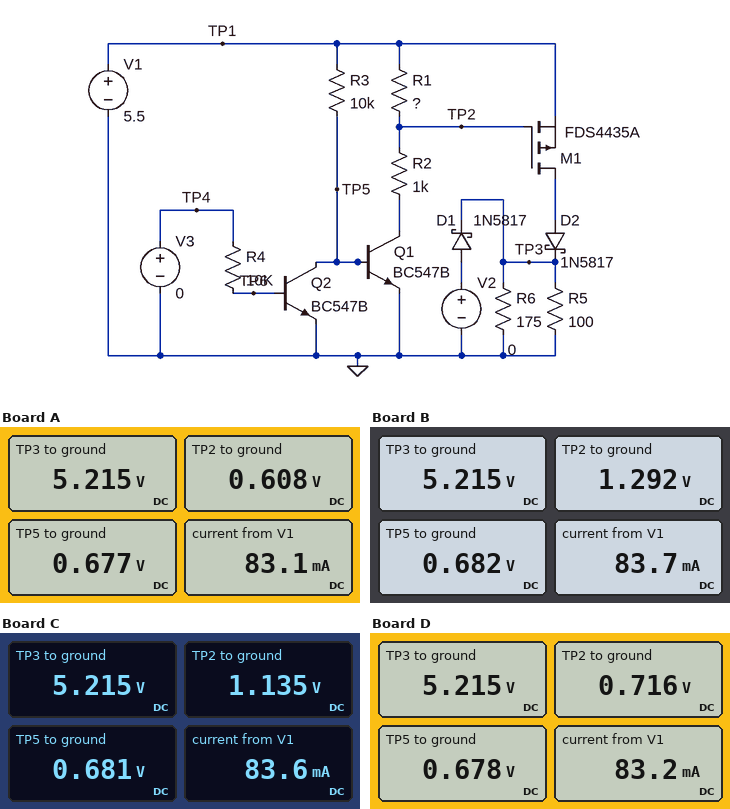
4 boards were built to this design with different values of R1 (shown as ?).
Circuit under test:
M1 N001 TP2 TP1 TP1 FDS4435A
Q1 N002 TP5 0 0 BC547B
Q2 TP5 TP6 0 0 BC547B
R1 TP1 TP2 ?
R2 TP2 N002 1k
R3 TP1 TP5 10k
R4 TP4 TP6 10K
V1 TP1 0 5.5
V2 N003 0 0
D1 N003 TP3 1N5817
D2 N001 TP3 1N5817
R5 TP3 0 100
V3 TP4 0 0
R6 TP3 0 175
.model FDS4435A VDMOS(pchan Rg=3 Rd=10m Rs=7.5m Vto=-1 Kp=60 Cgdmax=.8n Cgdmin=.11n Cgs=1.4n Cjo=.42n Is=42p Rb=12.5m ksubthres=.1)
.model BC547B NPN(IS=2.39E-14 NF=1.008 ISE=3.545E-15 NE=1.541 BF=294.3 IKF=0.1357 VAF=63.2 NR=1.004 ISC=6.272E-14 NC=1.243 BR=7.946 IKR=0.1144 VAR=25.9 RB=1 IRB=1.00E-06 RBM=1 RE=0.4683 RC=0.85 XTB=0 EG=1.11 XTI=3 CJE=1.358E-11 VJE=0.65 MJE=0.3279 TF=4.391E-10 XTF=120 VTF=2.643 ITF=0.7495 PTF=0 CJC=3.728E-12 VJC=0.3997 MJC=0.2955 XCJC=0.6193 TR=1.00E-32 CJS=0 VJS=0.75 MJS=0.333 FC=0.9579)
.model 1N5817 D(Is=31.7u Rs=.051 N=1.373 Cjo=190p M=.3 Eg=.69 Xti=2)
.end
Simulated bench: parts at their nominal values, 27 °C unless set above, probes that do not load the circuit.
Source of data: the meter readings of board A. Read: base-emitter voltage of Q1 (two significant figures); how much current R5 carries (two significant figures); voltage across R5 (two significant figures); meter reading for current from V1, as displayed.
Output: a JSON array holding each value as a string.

["680 mV", "52 mA", "5.2 V", "83.1 mA"]
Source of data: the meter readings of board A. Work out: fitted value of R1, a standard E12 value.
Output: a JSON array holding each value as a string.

["8.2 kΩ"]
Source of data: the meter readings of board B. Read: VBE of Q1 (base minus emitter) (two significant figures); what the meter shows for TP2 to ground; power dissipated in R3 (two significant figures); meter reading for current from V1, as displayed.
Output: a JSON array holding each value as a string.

["680 mV", "1.292 V", "2.3 mW", "83.7 mA"]
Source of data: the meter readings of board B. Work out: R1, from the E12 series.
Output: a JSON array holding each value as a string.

["3.3 kΩ"]
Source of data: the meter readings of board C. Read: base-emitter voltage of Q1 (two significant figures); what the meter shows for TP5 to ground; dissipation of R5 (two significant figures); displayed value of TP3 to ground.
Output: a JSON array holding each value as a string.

["680 mV", "0.681 V", "270 mW", "5.215 V"]
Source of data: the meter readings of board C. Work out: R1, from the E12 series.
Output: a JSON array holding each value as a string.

["3.9 kΩ"]
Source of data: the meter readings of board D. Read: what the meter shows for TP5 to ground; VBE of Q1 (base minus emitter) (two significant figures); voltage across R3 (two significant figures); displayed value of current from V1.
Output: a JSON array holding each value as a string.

["0.678 V", "680 mV", "4.8 V", "83.2 mA"]
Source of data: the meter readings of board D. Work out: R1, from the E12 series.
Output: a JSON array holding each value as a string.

["6.8 kΩ"]
